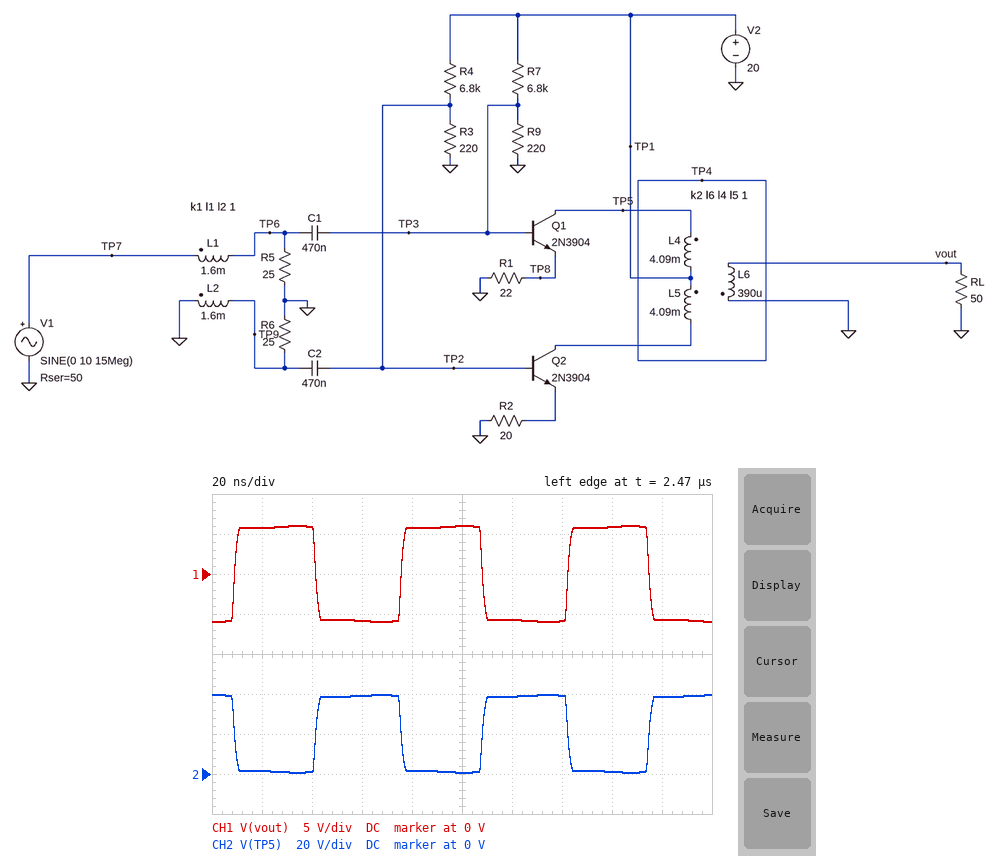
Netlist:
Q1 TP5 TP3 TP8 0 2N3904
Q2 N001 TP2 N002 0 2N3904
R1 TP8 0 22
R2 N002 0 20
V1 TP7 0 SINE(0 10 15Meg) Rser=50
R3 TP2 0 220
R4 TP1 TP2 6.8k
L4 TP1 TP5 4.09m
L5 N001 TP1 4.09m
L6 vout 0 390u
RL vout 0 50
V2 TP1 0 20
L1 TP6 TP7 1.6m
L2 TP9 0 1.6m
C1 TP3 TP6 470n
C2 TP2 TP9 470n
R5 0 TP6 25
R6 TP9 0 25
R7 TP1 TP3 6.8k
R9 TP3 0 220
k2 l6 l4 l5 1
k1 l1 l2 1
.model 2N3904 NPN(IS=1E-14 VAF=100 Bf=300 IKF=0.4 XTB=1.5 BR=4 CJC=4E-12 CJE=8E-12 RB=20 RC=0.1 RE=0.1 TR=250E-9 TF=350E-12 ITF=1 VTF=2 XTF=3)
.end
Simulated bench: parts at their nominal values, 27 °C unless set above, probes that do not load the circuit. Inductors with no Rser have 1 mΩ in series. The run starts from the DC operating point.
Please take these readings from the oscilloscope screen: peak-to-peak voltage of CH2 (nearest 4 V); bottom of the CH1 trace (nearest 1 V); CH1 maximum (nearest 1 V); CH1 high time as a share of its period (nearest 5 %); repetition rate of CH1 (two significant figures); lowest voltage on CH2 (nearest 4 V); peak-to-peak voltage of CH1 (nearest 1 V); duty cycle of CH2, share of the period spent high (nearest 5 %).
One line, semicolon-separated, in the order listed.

40 V; -6 V; 6 V; 50 %; 15 MHz; 0 V; 12 V; 50 %
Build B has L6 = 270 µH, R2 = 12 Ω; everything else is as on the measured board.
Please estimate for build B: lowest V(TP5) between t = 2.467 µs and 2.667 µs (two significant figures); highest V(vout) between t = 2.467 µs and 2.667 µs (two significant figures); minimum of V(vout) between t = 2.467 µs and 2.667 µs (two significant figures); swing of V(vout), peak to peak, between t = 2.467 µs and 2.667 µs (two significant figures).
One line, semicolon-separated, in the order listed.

320 mV; 5.1 V; -5.1 V; 10 V
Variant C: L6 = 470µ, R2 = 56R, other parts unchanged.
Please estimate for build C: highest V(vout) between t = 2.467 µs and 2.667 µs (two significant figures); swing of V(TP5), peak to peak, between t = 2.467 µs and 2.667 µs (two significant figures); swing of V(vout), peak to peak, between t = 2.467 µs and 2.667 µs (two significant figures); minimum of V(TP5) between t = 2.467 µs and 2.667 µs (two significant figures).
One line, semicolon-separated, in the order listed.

6.6 V; 37 V; 13 V; 600 mV
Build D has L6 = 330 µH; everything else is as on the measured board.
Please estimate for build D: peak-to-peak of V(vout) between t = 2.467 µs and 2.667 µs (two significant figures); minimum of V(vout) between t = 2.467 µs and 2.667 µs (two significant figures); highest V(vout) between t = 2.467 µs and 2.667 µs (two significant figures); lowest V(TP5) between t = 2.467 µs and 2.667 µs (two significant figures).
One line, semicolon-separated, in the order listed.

11 V; -5.6 V; 5.6 V; 420 mV
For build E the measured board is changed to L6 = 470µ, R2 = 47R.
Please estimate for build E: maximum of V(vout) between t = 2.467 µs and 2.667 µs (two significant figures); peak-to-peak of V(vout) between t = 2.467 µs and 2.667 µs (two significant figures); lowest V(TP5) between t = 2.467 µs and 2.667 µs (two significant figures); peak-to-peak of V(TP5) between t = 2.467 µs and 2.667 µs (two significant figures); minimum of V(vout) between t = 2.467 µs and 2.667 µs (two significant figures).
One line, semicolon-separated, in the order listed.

6.6 V; 13 V; 630 mV; 38 V; -6.3 V
